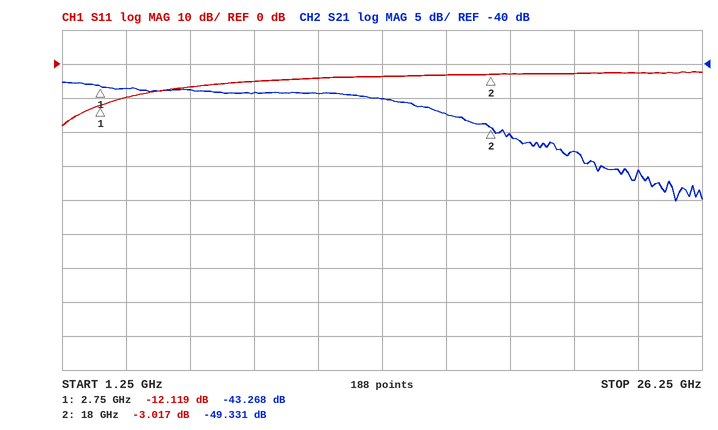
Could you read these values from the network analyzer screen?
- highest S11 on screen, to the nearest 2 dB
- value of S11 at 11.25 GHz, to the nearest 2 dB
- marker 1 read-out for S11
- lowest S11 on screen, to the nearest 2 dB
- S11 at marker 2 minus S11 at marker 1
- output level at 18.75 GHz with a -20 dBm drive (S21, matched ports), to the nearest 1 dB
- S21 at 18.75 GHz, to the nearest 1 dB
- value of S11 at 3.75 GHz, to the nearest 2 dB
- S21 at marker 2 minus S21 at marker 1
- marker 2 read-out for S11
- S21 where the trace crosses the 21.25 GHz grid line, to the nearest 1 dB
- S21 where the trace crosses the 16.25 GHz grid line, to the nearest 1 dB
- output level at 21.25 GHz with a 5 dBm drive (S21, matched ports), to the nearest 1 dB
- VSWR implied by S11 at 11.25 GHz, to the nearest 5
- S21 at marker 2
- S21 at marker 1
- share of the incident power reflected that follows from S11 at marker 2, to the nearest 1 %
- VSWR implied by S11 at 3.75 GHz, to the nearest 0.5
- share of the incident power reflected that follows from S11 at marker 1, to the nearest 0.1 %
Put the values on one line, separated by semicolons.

-2 dB; -4 dB; -12.119 dB; -18 dB; 9.102 dB; -70 dBm; -50 dB; -10 dB; -6.063 dB; -3.017 dB; -53 dB; -47 dB; -48 dBm; 5; -49.331 dB; -43.268 dB; 50 %; 2.0; 6.1 %
